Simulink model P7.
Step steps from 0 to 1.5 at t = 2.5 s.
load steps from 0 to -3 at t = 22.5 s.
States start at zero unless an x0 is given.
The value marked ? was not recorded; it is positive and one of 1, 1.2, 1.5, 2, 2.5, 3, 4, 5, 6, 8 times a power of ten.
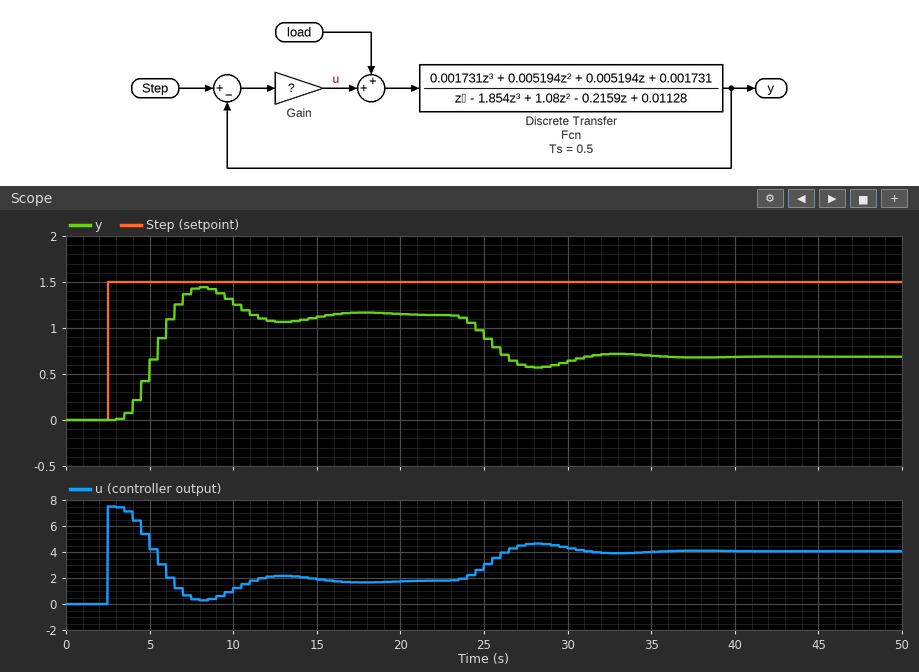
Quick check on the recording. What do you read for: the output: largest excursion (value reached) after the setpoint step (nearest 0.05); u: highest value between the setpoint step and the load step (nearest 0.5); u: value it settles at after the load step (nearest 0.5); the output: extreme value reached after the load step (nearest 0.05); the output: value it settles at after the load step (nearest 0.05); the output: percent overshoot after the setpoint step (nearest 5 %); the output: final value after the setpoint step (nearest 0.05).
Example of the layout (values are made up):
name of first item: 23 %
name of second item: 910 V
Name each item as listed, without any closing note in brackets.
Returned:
the output: largest excursion (value reached) after the setpoint step: 1.45
u: highest value between the setpoint step and the load step: 7.5
u: value it settles at after the load step: 4.0
the output: extreme value reached after the load step: 0.55
the output: value it settles at after the load step: 0.70
the output: percent overshoot after the setpoint step: 25 %
the output: final value after the setpoint step: 1.15
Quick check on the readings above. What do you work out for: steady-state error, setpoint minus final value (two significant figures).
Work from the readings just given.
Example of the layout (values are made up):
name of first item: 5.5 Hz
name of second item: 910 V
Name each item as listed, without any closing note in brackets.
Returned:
steady-state error, setpoint minus final value: 0.35
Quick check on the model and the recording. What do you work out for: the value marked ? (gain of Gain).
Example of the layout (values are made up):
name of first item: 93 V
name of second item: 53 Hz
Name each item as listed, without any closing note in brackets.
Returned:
the value marked ?: 5
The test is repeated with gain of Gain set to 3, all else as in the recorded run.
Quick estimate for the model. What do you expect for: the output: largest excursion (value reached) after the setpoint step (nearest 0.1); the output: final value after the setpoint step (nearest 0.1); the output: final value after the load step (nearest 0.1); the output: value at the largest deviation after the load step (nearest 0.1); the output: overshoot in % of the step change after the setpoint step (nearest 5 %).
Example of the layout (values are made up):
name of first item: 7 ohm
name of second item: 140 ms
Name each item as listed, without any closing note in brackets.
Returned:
the output: largest excursion (value reached) after the setpoint step: 1.1
the output: final value after the setpoint step: 1.0
the output: final value after the load step: 0.3
the output: value at the largest deviation after the load step: 0.3
the output: overshoot in % of the step change after the setpoint step: 10 %
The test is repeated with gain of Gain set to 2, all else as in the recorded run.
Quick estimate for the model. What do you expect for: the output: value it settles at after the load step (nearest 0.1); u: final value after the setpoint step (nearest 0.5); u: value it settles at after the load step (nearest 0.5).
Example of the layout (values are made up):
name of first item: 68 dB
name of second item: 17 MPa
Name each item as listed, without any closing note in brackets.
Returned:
the output: value it settles at after the load step: 0.0
u: final value after the setpoint step: 1.5
u: value it settles at after the load step: 3.0
